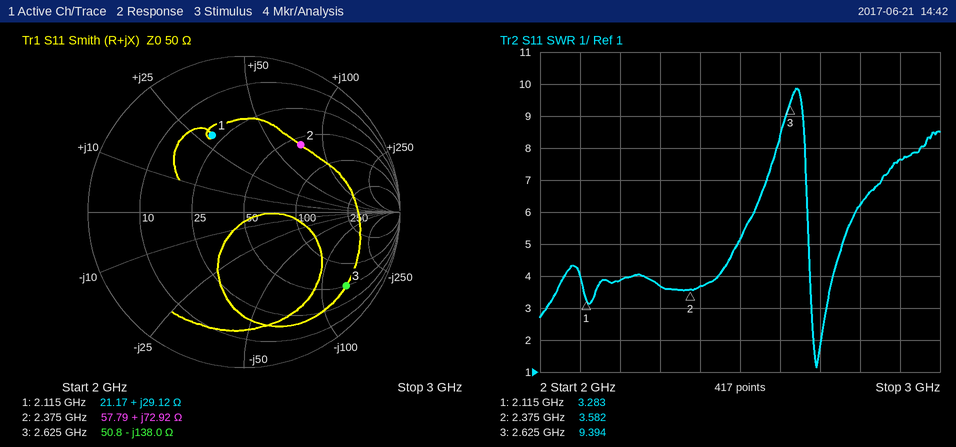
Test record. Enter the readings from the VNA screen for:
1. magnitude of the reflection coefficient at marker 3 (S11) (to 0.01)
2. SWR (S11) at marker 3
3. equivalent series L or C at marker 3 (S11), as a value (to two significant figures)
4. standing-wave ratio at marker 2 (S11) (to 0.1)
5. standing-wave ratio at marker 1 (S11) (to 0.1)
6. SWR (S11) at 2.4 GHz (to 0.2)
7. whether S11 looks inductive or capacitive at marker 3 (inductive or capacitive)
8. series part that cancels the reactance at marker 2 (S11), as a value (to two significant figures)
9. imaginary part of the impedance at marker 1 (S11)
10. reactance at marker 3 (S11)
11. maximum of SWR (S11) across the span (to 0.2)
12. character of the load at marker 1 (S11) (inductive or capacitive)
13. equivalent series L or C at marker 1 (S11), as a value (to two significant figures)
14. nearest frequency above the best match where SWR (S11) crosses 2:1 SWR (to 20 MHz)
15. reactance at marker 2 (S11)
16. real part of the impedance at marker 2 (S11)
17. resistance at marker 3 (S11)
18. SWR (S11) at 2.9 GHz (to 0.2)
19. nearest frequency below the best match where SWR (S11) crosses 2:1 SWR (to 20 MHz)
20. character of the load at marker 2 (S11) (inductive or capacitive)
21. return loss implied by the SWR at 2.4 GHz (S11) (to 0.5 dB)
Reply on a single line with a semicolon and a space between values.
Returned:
0.81; 9.394; 440 fF; 3.6; 3.3; 3.6; capacitive; 920 fF; +29.12 Ω; -138.0 Ω; 9.8; inductive; 2.2 nH; 2.70 GHz; +72.92 Ω; 57.79 Ω; 50.8 Ω; 7.6; 2.68 GHz; inductive; 5.0 dB
